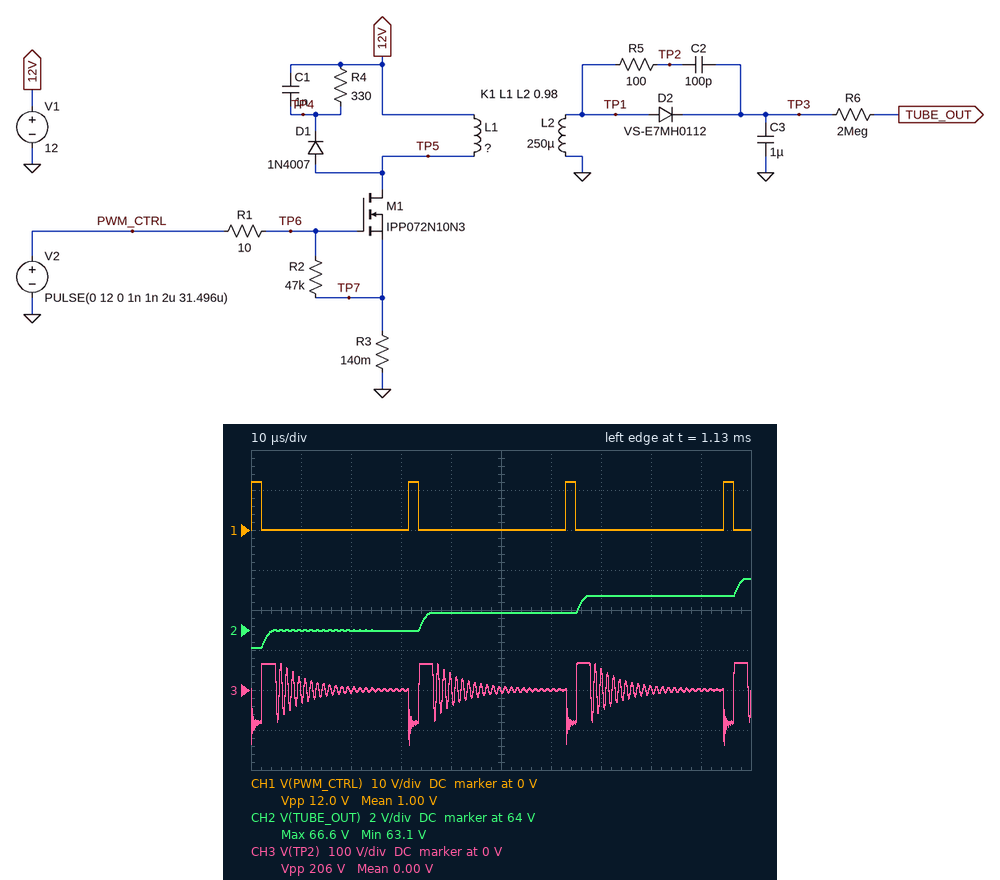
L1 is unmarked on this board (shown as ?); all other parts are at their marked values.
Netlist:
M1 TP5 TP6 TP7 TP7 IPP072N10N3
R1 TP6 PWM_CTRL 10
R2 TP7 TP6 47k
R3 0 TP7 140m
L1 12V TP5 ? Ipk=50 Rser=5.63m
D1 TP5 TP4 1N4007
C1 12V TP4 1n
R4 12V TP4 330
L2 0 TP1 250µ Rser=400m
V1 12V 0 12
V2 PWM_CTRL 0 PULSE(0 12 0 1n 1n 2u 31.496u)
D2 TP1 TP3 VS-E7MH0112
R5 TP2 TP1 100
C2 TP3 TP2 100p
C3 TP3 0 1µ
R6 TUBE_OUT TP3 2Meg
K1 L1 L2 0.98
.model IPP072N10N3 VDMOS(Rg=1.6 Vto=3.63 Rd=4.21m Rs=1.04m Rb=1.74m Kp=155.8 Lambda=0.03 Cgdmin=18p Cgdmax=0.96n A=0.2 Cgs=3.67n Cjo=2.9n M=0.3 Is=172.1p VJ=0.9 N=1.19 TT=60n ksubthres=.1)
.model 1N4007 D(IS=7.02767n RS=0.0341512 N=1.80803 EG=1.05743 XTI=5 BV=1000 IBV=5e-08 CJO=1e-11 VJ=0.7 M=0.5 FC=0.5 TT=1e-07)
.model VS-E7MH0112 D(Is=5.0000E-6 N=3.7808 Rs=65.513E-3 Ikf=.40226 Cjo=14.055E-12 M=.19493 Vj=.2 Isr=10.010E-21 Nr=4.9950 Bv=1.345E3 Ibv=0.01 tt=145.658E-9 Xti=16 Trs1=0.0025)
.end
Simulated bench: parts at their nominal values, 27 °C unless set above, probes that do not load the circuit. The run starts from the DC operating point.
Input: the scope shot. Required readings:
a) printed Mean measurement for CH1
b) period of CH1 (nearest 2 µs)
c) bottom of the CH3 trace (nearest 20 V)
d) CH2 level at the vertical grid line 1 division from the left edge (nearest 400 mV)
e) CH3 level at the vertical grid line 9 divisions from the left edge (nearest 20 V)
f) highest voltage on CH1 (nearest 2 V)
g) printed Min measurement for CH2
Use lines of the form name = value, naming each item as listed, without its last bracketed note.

printed Mean measurement for CH1 = 1.00 V
period of CH1 = 32 µs
bottom of the CH3 trace = -140 V
CH2 level at the vertical grid line 1 division from the left edge = 64.0 V
CH3 level at the vertical grid line 9 divisions from the left edge = 0 V
highest voltage on CH1 = 12 V
printed Min measurement for CH2 = 63.1 V
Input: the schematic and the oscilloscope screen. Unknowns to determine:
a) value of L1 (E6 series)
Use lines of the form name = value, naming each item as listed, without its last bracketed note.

value of L1 = 4.7 µH
